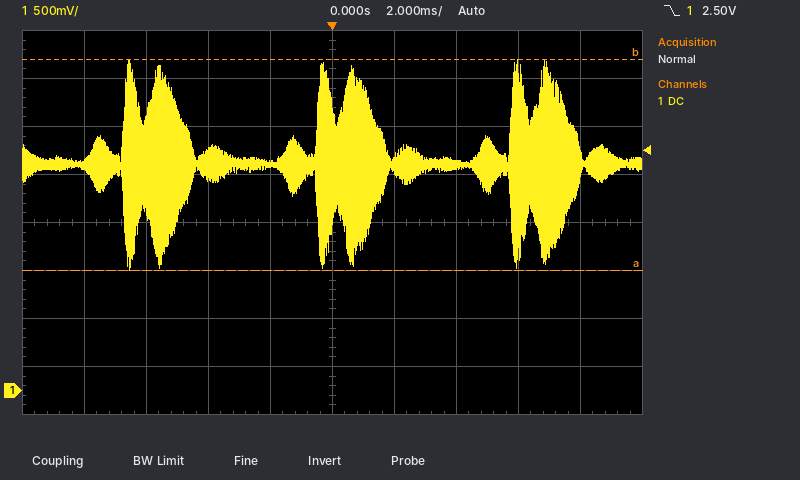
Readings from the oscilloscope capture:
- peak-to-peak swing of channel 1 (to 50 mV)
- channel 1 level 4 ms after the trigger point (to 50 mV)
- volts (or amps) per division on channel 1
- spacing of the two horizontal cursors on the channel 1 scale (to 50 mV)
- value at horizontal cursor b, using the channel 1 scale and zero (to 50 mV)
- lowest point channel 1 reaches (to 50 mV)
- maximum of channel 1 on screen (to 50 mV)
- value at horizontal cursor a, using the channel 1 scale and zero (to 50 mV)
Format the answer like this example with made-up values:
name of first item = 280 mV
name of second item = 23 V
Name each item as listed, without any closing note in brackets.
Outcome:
peak-to-peak swing of channel 1 = 2.20 V
channel 1 level 4 ms after the trigger point = 2.35 V
volts (or amps) per division on channel 1 = 500 mV
spacing of the two horizontal cursors on the channel 1 scale = 2.20 V
value at horizontal cursor b, using the channel 1 scale and zero = 3.45 V
lowest point channel 1 reaches = 1.25 V
maximum of channel 1 on screen = 3.45 V
value at horizontal cursor a, using the channel 1 scale and zero = 1.25 V
